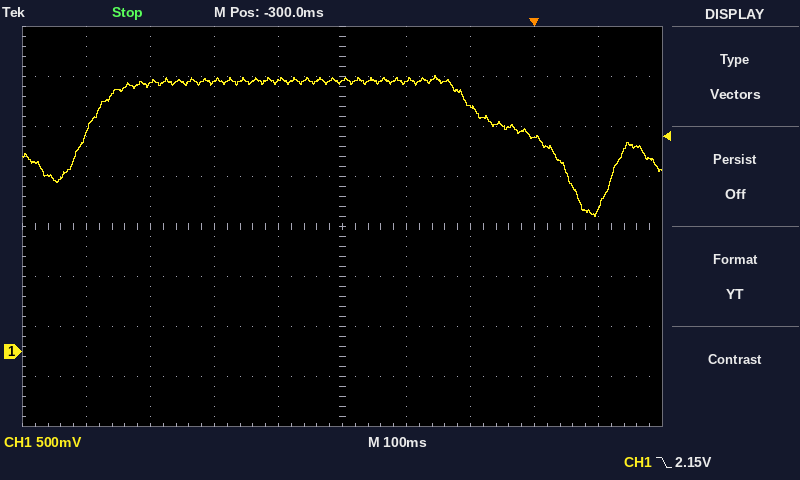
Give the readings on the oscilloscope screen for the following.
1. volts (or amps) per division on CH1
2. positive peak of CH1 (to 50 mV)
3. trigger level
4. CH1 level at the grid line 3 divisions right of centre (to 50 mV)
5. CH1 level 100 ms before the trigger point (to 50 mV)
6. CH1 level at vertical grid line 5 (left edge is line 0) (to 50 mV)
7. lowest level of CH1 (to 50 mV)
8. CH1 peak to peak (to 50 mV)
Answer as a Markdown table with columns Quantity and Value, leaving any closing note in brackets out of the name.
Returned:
| Quantity | Value |
|---|---|
| volts (or amps) per division on CH1 | 500 mV |
| positive peak of CH1 | 2.75 V |
| trigger level | 2.15 V |
| CH1 level at the grid line 3 divisions right of centre | 2.15 V |
| CH1 level 100 ms before the trigger point | 2.45 V |
| CH1 level at vertical grid line 5 (left edge is line 0) | 2.70 V |
| lowest level of CH1 | 1.35 V |
| CH1 peak to peak | 1.40 V |
